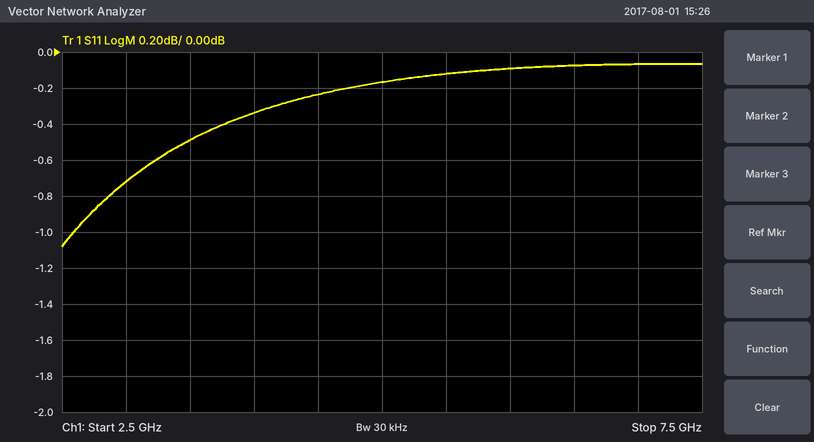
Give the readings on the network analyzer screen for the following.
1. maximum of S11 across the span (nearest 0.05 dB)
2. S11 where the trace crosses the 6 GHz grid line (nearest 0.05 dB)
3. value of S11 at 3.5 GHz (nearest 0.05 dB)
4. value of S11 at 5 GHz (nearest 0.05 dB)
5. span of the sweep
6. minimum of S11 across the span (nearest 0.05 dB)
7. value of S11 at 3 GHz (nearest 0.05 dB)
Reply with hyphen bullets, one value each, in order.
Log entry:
- -0.05 dB
- -0.10 dB
- -0.50 dB
- -0.15 dB
- 5 GHz
- -1.10 dB
- -0.70 dB
